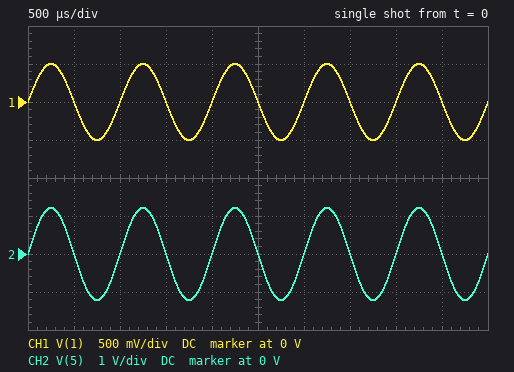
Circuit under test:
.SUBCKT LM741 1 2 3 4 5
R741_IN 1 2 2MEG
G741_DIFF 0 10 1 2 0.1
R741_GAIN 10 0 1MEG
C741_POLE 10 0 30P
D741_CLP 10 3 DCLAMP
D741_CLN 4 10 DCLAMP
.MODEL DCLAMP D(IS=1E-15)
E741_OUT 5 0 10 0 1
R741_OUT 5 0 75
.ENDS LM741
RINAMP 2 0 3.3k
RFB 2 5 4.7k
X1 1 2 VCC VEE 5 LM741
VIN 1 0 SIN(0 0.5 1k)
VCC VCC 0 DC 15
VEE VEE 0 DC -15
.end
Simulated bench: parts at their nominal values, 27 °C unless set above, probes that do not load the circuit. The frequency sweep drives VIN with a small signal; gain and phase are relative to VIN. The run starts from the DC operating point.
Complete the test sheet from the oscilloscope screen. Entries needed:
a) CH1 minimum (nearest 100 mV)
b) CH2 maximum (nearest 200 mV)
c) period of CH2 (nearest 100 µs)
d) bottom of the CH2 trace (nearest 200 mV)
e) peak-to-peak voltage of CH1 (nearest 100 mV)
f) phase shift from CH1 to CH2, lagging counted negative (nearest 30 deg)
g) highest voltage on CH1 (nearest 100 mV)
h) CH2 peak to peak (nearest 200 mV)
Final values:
-500 mV
1.2 V
1.0 ms
-1.2 V
1.0 V
0 deg
500 mV
2.4 V
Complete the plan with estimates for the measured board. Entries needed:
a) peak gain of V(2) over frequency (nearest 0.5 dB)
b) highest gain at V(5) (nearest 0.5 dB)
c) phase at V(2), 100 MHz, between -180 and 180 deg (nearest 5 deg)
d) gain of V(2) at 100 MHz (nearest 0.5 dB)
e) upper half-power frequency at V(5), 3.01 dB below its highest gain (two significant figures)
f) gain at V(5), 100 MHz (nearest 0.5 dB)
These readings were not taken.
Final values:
0 dB
7.5 dB
-25 deg
-1.0 dB
220 MHz
7.0 dB
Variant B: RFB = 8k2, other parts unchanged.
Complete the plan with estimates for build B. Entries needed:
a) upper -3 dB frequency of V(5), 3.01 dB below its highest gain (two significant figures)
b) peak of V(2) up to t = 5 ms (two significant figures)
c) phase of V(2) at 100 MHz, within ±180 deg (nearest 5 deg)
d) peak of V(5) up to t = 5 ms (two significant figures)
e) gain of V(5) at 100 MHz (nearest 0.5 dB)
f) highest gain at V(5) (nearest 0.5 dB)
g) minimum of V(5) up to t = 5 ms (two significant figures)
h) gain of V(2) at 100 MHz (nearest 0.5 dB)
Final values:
150 MHz
500 mV
-35 deg
1.7 V
9.5 dB
11.0 dB
-1.7 V
-1.5 dB
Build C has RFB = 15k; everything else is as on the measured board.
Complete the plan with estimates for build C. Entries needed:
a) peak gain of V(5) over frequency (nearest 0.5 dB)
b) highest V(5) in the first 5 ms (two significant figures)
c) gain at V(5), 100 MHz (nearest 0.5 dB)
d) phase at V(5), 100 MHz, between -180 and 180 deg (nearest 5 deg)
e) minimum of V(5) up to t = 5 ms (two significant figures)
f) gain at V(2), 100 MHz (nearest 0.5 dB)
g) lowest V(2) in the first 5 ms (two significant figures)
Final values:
15.0 dB
2.8 V
11.5 dB
-45 deg
-2.8 V
-3.0 dB
-500 mV
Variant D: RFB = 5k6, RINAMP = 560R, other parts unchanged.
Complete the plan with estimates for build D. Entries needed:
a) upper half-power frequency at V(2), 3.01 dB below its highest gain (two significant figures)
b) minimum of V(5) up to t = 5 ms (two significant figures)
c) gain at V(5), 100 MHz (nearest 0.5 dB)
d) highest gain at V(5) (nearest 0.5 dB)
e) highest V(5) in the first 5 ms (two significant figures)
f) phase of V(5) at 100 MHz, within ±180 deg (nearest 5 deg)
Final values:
48 MHz
-5.5 V
13.5 dB
21.0 dB
5.5 V
-65 deg
